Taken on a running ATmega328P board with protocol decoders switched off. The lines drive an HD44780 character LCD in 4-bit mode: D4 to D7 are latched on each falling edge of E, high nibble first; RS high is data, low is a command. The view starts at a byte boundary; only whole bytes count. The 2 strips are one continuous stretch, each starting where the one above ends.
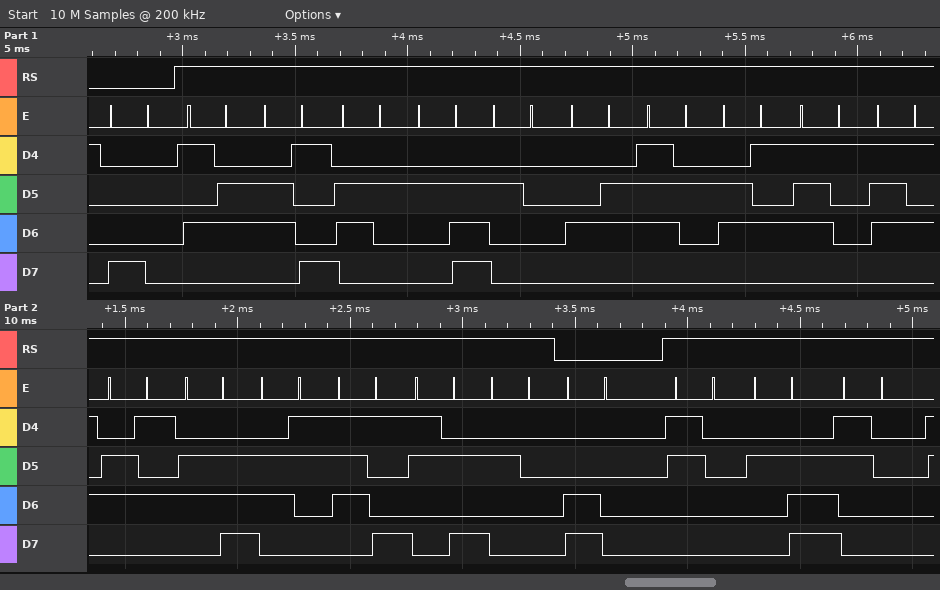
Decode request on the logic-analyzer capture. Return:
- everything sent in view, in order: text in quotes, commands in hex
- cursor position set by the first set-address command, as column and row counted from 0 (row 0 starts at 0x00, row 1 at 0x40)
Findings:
0x80 "Vib. Frequency: " 0xC0 "0.0"
column 0, row 0
